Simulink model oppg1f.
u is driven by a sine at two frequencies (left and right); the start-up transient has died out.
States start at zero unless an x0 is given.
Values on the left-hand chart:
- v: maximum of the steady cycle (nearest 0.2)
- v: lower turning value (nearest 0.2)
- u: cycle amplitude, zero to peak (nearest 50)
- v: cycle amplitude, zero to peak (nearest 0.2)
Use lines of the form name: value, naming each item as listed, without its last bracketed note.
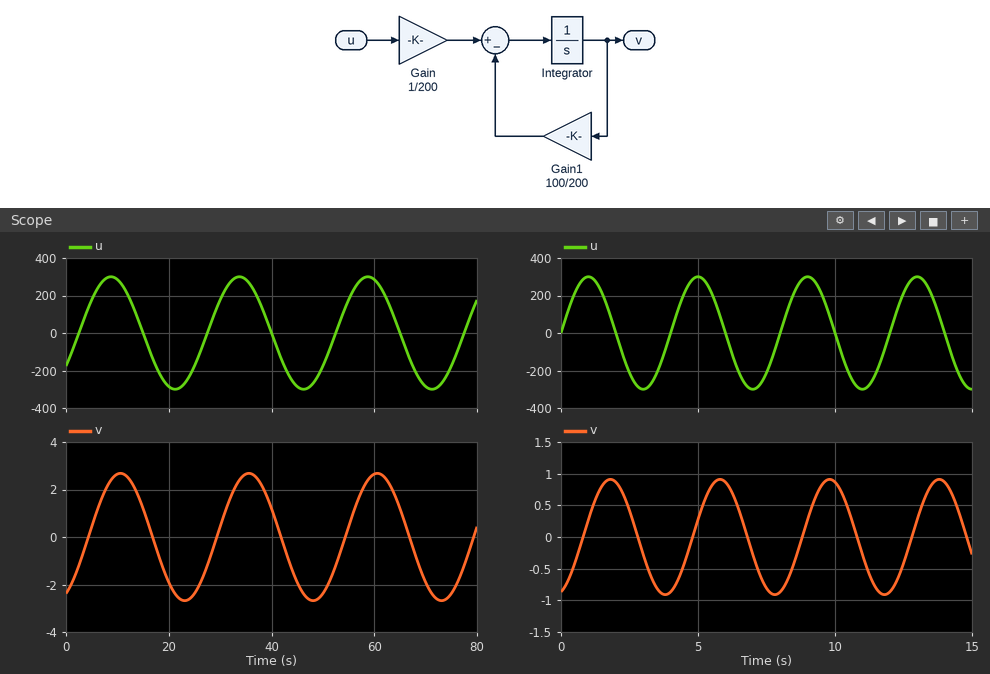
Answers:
v: maximum of the steady cycle: 2.6
v: lower turning value: -2.6
u: cycle amplitude, zero to peak: 300
v: cycle amplitude, zero to peak: 2.6
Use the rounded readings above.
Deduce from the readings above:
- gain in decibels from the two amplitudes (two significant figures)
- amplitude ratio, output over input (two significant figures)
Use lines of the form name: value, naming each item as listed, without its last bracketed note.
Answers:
gain in decibels from the two amplitudes: -41 dB
amplitude ratio, output over input: 0.0087
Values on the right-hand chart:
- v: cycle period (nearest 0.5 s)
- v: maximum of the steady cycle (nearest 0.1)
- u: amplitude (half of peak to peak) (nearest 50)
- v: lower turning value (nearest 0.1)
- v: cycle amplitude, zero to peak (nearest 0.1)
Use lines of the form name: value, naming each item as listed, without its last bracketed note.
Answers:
v: cycle period: 4.0 s
v: maximum of the steady cycle: 0.9
u: amplitude (half of peak to peak): 300
v: lower turning value: -0.9
v: cycle amplitude, zero to peak: 0.9
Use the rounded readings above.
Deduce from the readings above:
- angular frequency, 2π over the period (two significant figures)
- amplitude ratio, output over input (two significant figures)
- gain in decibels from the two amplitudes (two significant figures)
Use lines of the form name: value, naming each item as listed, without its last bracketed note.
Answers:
angular frequency, 2π over the period: 1.6 rad/s
amplitude ratio, output over input: 0.0030
gain in decibels from the two amplitudes: -50 dB
